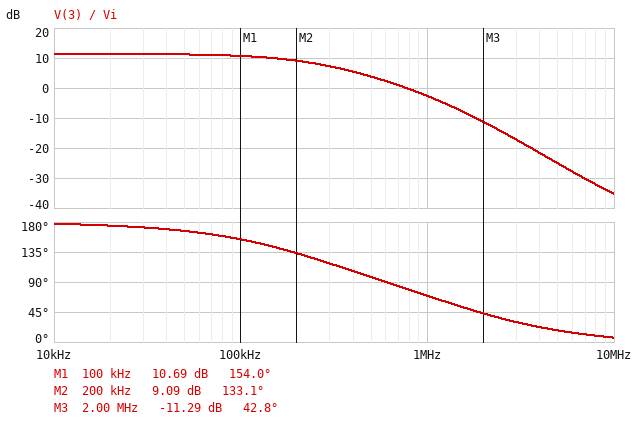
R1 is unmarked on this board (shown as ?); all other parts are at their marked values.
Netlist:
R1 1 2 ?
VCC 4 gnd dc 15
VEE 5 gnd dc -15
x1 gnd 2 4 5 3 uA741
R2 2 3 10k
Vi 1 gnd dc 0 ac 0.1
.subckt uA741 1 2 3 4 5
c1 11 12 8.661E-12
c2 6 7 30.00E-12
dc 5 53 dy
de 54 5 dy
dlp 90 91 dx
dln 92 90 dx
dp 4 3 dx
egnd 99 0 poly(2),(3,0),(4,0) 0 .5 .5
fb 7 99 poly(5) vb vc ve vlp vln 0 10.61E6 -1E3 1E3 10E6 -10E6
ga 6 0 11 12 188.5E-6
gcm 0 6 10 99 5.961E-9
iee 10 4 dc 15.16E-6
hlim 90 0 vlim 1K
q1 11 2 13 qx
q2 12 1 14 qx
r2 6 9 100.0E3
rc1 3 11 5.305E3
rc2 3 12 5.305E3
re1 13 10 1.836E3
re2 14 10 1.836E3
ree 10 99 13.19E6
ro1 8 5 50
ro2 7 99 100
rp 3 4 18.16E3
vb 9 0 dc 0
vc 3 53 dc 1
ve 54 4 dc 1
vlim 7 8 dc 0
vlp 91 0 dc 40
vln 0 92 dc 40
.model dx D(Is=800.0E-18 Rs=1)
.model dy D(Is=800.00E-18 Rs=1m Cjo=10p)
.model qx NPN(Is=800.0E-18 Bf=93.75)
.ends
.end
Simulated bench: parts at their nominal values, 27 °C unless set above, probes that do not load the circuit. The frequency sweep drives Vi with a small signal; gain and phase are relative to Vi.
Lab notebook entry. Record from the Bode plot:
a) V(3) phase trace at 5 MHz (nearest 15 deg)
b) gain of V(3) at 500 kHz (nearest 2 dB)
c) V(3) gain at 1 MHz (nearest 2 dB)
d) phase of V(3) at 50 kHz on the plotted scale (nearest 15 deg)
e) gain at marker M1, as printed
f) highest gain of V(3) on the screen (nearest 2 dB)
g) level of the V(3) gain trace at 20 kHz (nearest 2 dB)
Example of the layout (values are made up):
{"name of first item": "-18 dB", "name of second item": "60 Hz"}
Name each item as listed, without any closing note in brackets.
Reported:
{"V(3) phase trace at 5 MHz": "15 deg", "gain of V(3) at 500 kHz": "4 dB", "V(3) gain at 1 MHz": "-2 dB", "phase of V(3) at 50 kHz on the plotted scale": "165 deg", "gain at marker M1, as printed": "10.69 dB", "highest gain of V(3) on the screen": "12 dB", "level of the V(3) gain trace at 20 kHz": "12 dB"}
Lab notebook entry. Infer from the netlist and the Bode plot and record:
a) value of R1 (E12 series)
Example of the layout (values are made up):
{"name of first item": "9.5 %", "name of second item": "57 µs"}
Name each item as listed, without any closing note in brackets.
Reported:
{"value of R1": "2.7 kΩ"}
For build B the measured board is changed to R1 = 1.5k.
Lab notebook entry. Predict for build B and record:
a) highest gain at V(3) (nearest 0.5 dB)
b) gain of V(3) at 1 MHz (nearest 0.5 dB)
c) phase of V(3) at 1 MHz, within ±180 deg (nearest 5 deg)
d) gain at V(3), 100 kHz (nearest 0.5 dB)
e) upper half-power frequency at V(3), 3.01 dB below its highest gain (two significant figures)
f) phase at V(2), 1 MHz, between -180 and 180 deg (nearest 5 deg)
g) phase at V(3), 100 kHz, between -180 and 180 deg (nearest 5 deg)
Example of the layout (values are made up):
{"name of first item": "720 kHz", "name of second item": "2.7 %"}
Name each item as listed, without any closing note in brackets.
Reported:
{"highest gain at V(3)": "16.5 dB", "gain of V(3) at 1 MHz": "-2.0 dB", "phase of V(3) at 1 MHz, within ±180 deg": "65 deg", "gain at V(3), 100 kHz": "14.5 dB", "upper half-power frequency at V(3), 3.01 dB below its highest gain": "140 kHz", "phase at V(2), 1 MHz, between -180 and 180 deg": "5 deg", "phase at V(3), 100 kHz, between -180 and 180 deg": "140 deg"}
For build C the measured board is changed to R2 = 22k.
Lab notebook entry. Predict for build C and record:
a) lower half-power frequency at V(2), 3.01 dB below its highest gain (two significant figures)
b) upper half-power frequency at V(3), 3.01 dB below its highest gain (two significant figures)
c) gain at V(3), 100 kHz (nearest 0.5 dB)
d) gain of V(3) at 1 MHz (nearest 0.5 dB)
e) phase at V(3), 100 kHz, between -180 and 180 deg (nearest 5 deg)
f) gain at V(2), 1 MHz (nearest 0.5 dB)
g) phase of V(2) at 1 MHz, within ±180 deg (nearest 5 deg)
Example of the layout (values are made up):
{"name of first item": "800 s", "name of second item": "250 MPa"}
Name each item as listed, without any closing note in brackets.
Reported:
{"lower half-power frequency at V(2), 3.01 dB below its highest gain": "110 kHz", "upper half-power frequency at V(3), 3.01 dB below its highest gain": "120 kHz", "gain at V(3), 100 kHz": "16.0 dB", "gain of V(3) at 1 MHz": "-2.0 dB", "phase at V(3), 100 kHz, between -180 and 180 deg": "135 deg", "gain at V(2), 1 MHz": "-0.5 dB", "phase of V(2) at 1 MHz, within ±180 deg": "5 deg"}
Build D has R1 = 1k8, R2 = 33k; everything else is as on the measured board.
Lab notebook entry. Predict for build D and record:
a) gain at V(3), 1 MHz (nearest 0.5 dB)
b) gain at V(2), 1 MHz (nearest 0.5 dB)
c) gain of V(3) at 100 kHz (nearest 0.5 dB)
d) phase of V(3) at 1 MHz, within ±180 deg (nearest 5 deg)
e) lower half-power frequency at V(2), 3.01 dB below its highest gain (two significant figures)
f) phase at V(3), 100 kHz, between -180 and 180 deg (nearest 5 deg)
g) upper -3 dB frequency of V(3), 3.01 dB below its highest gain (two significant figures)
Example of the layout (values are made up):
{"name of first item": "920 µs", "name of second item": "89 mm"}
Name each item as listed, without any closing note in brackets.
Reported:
{"gain at V(3), 1 MHz": "-1.5 dB", "gain at V(2), 1 MHz": "-0.5 dB", "gain of V(3) at 100 kHz": "18.5 dB", "phase of V(3) at 1 MHz, within ±180 deg": "60 deg", "lower half-power frequency at V(2), 3.01 dB below its highest gain": "52 kHz", "phase at V(3), 100 kHz, between -180 and 180 deg": "115 deg", "upper -3 dB frequency of V(3), 3.01 dB below its highest gain": "53 kHz"}
